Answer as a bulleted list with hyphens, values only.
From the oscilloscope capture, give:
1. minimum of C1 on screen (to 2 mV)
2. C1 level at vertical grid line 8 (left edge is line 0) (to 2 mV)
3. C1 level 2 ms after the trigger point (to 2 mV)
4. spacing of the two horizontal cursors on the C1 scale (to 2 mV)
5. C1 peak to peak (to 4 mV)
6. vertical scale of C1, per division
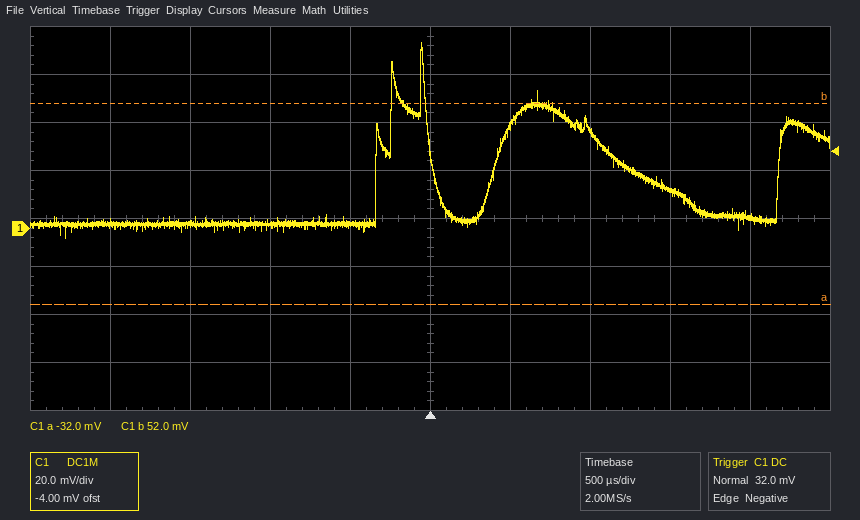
- -4 mV
- 16 mV
- 4 mV
- 84 mV
- 80 mV
- 20 mV
